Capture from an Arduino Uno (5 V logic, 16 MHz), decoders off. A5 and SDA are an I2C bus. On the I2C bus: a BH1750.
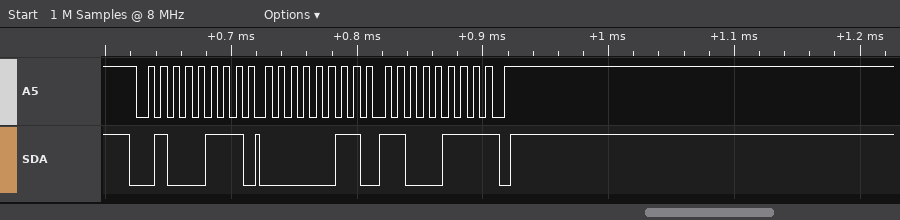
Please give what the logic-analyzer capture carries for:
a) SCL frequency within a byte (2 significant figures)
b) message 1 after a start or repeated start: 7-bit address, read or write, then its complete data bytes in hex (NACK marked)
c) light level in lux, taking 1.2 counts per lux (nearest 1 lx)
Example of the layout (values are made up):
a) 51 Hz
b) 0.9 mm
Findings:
a) 100 kHz
b) 0x23 read: 03 C7 NACK
c) 806 lx
